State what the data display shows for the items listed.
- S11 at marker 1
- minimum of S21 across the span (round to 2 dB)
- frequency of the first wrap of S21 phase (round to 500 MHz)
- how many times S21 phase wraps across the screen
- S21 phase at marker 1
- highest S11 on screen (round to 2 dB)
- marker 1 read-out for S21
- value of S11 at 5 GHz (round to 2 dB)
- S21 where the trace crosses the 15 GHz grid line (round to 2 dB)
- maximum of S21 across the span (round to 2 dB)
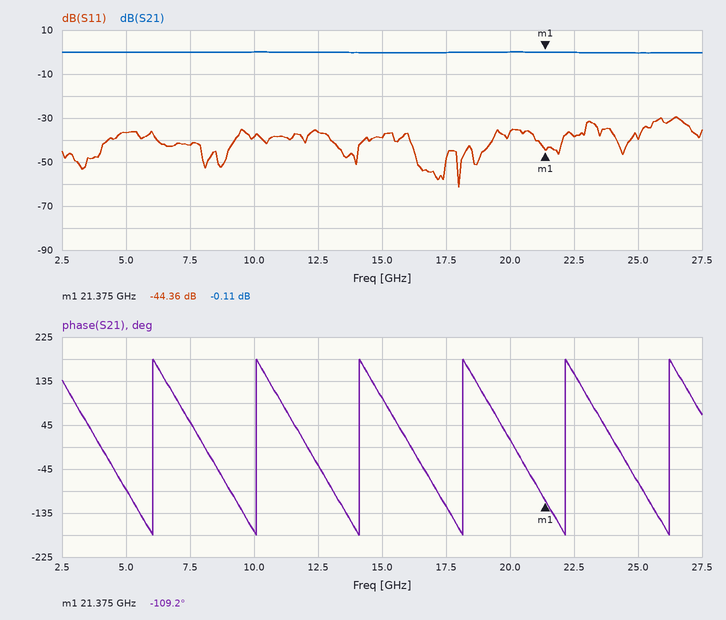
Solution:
-44.36 dB
0 dB
6.0 GHz
6
-109.2°
-30 dB
-0.11 dB
-36 dB
0 dB
0 dB
